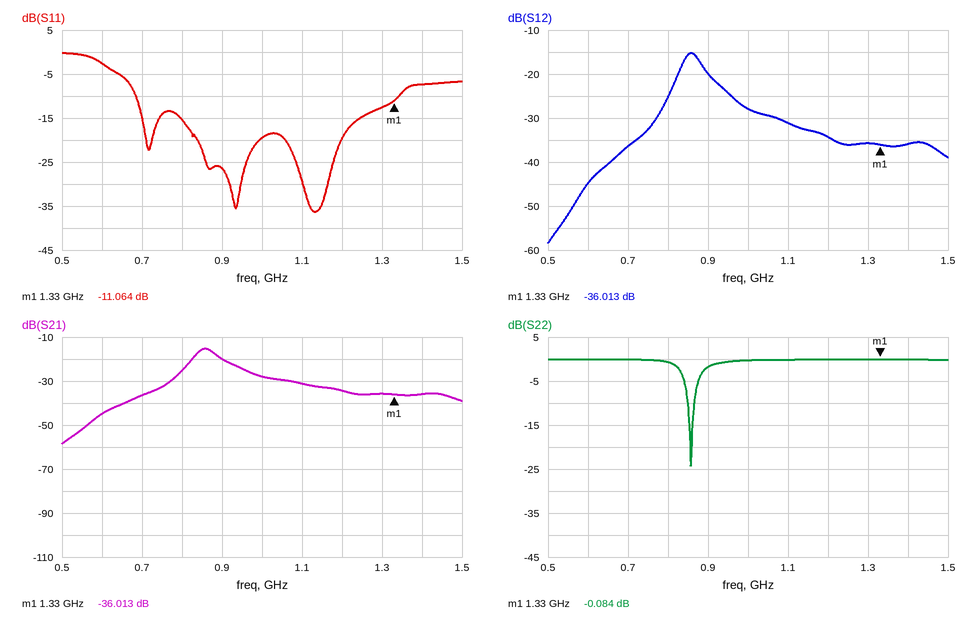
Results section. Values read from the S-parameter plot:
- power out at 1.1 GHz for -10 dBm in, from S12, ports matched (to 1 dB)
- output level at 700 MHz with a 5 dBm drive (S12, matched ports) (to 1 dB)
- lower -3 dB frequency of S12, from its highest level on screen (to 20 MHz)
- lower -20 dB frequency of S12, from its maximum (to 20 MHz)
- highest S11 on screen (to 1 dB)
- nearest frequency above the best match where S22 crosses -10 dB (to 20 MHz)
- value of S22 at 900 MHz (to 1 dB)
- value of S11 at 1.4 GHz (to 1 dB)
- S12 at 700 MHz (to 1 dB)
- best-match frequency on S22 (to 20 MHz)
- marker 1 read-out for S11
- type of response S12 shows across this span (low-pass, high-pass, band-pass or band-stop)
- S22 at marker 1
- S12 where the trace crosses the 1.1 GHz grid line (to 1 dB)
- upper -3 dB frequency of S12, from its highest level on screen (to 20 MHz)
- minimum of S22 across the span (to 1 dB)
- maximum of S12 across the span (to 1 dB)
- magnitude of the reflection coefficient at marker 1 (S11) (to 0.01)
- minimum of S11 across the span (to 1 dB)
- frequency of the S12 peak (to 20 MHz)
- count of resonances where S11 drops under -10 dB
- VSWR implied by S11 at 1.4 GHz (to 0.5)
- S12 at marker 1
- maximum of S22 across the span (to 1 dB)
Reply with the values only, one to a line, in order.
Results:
-41 dBm
-31 dBm
840 MHz
720 MHz
0 dB
860 MHz
-2 dB
-7 dB
-36 dB
860 MHz
-11.064 dB
band-pass
-0.084 dB
-31 dB
880 MHz
-24 dB
-15 dB
0.28
-36 dB
860 MHz
3
2.5
-36.013 dB
0 dB
